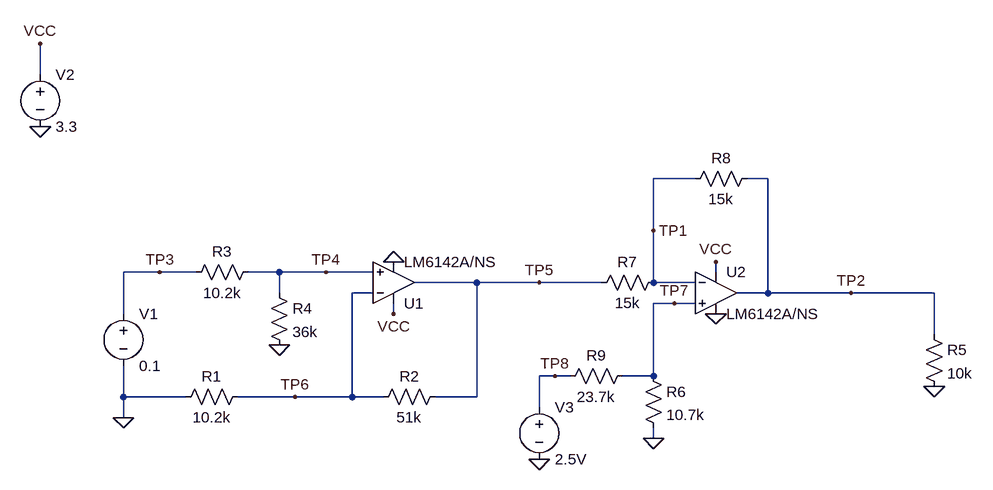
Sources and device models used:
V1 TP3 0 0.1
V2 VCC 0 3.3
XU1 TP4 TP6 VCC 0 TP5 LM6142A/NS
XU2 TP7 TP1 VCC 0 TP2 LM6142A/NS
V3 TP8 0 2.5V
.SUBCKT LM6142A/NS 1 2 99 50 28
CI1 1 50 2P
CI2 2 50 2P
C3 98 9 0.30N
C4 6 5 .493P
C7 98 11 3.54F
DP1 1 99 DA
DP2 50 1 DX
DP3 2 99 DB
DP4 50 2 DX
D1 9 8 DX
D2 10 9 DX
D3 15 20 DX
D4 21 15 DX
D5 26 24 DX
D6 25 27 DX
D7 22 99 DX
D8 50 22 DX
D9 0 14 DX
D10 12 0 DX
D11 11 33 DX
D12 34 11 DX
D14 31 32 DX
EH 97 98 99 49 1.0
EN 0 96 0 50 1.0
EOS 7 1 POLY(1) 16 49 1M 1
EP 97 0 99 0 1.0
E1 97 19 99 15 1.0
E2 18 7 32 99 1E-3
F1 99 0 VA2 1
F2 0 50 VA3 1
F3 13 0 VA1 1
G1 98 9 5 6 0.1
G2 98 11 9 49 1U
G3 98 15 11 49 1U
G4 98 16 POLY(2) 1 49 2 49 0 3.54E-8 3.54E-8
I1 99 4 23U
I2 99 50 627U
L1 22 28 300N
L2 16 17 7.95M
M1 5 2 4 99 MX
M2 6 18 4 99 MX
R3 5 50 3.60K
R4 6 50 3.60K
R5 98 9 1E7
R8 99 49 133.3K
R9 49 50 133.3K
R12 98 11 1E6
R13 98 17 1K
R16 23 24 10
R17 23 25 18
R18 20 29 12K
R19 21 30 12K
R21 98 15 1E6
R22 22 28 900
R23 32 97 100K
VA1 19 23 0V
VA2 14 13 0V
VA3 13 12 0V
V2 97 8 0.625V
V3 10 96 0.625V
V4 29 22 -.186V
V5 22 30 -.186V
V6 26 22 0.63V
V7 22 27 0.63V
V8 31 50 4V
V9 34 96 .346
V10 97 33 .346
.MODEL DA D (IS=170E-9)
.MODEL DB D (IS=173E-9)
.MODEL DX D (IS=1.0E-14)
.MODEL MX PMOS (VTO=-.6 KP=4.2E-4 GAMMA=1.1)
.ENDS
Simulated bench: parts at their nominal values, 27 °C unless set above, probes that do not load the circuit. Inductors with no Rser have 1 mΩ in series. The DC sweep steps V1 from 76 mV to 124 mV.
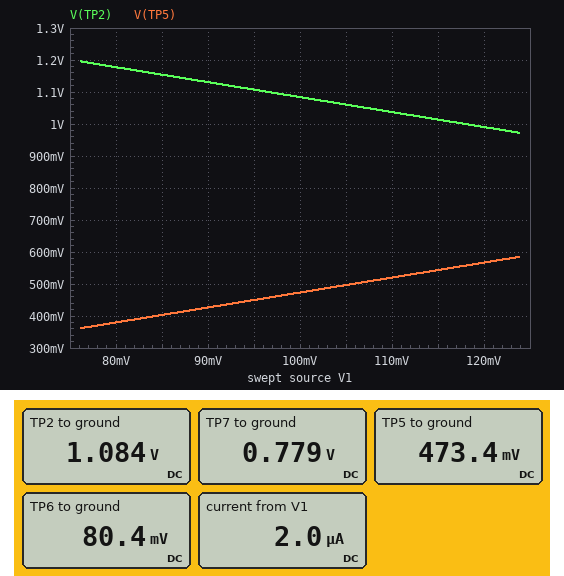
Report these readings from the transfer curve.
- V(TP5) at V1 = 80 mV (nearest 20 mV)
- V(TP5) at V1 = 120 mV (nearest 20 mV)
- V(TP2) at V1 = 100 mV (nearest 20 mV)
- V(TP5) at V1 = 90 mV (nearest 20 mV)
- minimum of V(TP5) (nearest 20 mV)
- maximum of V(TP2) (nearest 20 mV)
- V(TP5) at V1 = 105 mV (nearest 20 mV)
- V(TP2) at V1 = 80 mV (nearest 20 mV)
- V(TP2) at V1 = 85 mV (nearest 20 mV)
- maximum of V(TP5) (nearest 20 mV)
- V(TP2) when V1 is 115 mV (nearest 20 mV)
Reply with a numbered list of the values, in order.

1. 380 mV
2. 560 mV
3. 1.08 V
4. 420 mV
5. 360 mV
6. 1.20 V
7. 500 mV
8. 1.18 V
9. 1.16 V
10. 580 mV
11. 1.02 V
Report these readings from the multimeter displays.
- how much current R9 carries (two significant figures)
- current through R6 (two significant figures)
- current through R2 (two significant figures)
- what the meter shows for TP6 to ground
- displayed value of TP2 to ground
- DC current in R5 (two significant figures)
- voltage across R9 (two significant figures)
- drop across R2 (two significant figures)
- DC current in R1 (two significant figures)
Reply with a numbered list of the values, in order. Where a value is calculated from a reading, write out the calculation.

1. (2.5 V - 779 mV) / 23.7 kΩ = 73 µA
2. (779 mV) / 10.7 kΩ = 73 µA
3. (473.4 mV - 80.4 mV) / 51 kΩ = 7.7 µA
4. 80.4 mV
5. 1.084 V
6. (1.084 V) / 10 kΩ = 110 µA
7. 2.5 V - 779 mV = 1.7 V
8. 473.4 mV - 80.4 mV = 390 mV
9. (80.4 mV) / 10.2 kΩ = 7.9 µA
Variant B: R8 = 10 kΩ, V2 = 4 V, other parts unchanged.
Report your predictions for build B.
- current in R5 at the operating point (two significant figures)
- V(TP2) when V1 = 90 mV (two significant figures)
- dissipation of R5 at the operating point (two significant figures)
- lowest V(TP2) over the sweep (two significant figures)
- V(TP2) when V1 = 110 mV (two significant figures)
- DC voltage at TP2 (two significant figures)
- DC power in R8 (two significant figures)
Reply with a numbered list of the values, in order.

1. 98 µA
2. 1.0 V
3. 97 µW
4. 910 mV
5. 950 mV
6. 980 mV
7. 4.1 µW
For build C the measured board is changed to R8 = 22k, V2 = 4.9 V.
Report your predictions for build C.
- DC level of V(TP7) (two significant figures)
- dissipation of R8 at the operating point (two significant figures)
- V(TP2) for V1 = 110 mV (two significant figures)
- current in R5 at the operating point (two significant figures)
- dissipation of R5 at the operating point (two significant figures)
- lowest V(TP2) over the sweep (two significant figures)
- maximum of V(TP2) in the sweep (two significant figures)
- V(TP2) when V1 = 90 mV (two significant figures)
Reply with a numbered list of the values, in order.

1. 780 mV
2. 9.1 µW
3. 1.2 V
4. 120 µA
5. 150 µW
6. 1.1 V
7. 1.4 V
8. 1.3 V
